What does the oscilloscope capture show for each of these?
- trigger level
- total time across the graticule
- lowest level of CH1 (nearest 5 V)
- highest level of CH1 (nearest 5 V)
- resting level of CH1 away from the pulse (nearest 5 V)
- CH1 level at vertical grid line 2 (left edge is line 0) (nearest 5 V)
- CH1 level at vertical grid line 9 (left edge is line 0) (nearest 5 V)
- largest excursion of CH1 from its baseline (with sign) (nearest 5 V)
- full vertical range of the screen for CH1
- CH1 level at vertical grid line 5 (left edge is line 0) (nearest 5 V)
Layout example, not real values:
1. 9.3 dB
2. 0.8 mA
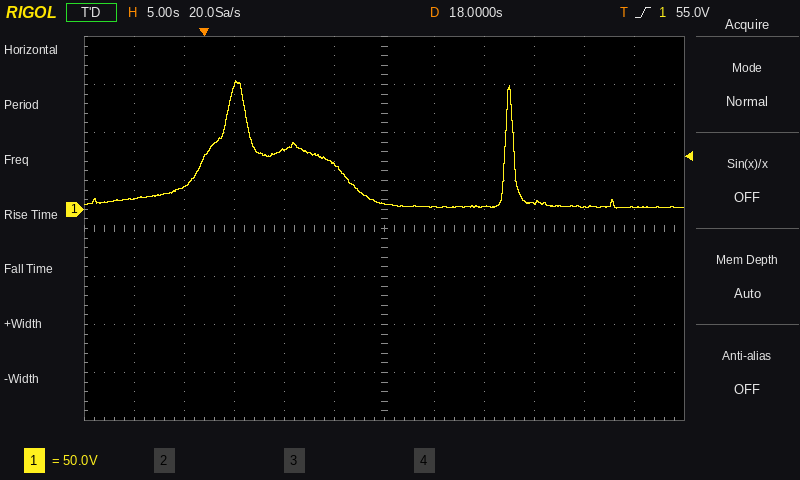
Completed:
1. 55.0 V
2. 60 s
3. 0 V
4. 135 V
5. 5 V
6. 25 V
7. 5 V
8. +130 V
9. 400 V
10. 45 V
